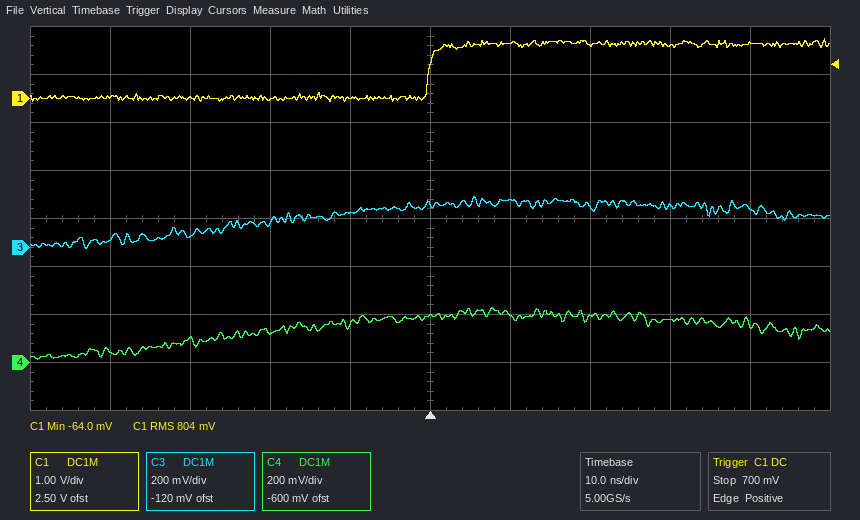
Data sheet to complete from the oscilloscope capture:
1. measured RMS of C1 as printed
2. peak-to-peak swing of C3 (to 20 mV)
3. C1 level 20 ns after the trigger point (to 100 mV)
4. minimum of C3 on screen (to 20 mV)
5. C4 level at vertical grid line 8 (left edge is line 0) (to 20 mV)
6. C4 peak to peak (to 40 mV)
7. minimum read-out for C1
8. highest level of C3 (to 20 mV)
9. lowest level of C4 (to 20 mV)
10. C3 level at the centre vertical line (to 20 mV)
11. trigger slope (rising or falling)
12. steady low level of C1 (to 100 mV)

804 mV
220 mV
1.1 V
0 mV
180 mV
200 mV
-64.0 mV
220 mV
20 mV
180 mV
rising
0.0 V
